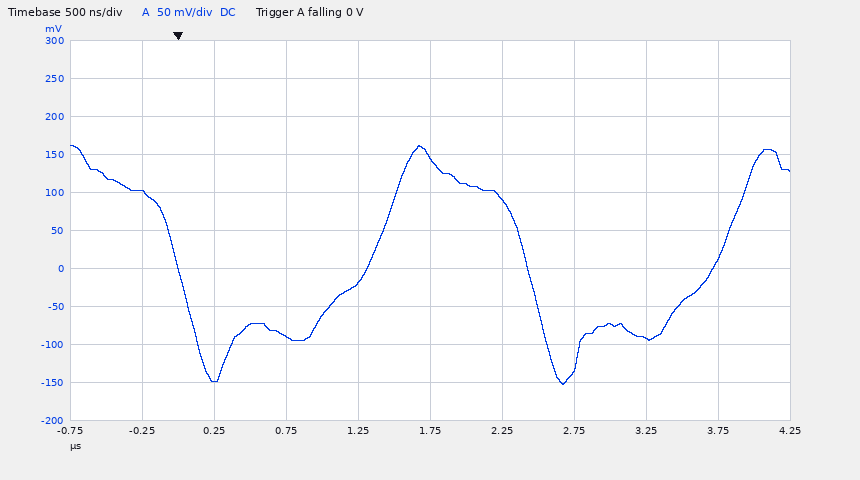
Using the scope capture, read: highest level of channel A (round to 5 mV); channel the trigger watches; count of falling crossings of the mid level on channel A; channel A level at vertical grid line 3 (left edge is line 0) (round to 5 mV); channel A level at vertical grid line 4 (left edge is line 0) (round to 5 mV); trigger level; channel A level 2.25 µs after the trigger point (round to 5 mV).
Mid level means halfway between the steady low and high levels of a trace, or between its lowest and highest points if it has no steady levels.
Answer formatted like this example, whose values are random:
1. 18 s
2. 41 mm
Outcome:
1. 160 mV
2. channel A
3. 2
4. -90 mV
5. -20 mV
6. 0 V
7. 90 mV
